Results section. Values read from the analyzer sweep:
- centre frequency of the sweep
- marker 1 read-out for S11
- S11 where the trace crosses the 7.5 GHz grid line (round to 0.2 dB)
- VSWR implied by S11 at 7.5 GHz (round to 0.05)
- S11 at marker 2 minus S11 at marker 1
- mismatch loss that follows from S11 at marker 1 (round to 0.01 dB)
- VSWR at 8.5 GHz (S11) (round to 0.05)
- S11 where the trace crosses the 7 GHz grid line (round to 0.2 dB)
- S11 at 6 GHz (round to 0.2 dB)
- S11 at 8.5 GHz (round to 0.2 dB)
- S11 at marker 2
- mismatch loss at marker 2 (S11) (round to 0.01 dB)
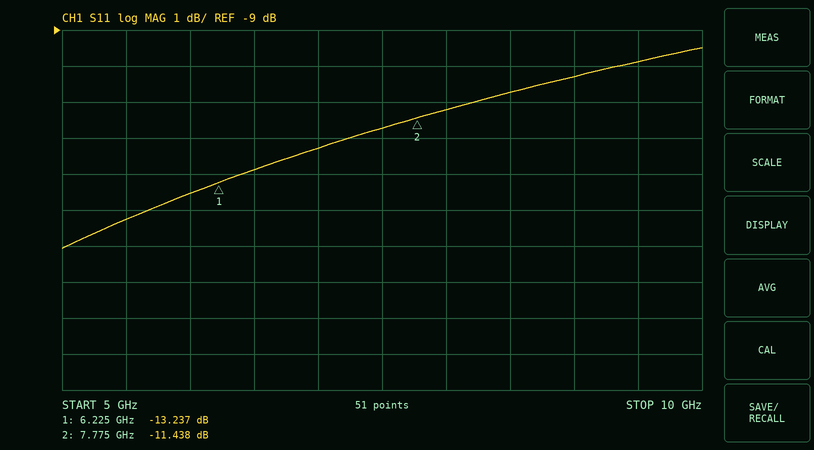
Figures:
7.5 GHz
-13.237 dB
-11.8 dB
1.70
1.799 dB
0.21 dB
1.80
-12.2 dB
-13.6 dB
-10.8 dB
-11.438 dB
0.32 dB
